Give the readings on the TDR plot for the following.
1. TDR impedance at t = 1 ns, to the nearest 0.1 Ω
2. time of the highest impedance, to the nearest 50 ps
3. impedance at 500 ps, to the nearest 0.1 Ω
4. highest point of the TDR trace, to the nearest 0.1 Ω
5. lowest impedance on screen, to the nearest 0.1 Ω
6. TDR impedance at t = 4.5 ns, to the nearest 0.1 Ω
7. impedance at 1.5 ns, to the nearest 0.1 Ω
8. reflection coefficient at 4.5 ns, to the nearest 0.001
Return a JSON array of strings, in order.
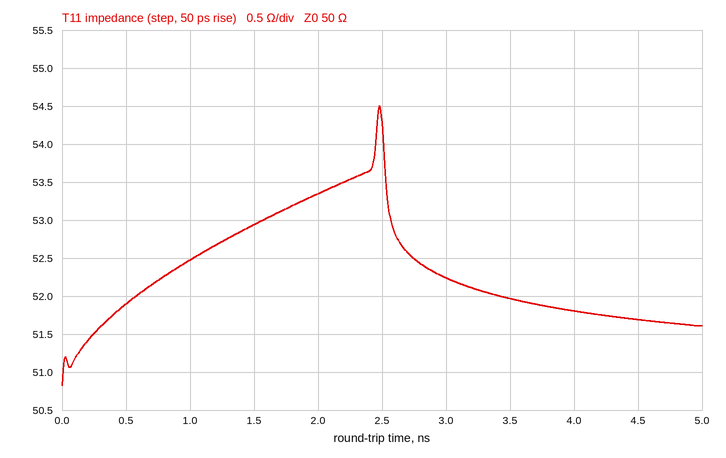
["52.5 Ω", "2.50 ns", "51.9 Ω", "54.5 Ω", "50.8 Ω", "51.7 Ω", "52.9 Ω", "+0.017"]
